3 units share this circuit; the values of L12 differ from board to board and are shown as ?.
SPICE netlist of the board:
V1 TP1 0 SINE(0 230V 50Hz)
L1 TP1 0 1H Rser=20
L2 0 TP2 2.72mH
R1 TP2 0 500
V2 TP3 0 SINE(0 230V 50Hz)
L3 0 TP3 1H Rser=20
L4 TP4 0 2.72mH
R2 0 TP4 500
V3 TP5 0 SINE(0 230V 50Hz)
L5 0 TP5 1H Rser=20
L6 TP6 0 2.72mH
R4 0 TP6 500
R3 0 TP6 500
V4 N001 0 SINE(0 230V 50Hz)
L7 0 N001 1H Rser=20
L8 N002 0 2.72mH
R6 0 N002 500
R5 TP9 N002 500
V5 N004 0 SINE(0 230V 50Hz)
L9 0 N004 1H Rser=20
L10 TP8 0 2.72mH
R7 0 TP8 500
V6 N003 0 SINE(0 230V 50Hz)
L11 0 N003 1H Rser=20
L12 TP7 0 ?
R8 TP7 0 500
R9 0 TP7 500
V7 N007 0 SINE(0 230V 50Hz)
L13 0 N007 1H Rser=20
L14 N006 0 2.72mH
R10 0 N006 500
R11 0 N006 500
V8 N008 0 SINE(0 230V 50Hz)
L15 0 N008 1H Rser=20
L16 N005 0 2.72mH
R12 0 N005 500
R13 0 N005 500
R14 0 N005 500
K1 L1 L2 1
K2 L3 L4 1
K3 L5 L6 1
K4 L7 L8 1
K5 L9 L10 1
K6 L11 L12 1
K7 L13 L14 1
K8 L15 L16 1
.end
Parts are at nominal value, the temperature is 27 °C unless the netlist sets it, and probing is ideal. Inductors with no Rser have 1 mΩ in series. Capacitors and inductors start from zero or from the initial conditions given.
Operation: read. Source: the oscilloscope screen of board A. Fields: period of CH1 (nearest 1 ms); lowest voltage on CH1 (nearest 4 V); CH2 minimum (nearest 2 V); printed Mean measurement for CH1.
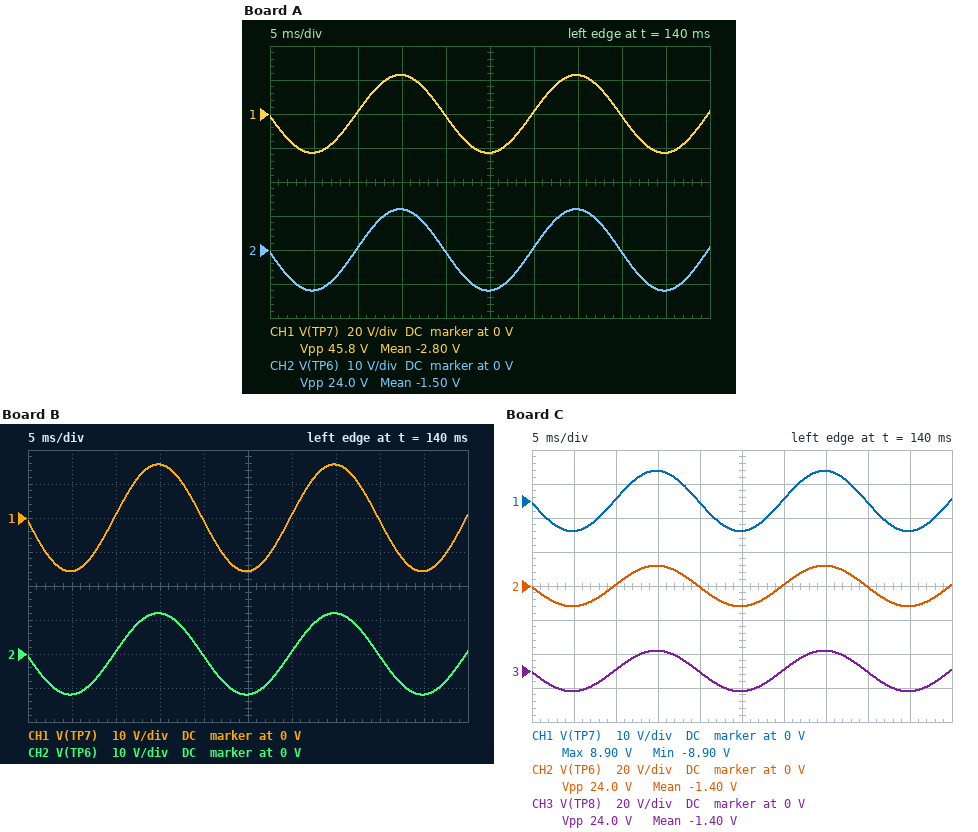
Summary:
20 ms
-24 V
-12 V
-2.80 V
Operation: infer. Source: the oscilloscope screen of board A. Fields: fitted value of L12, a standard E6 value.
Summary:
10 mH
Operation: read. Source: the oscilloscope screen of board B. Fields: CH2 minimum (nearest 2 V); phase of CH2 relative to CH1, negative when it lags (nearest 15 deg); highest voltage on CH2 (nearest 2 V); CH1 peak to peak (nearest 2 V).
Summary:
-12 V
0 deg
12 V
32 V
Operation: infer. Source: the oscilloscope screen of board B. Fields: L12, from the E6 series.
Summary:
4.7 mH
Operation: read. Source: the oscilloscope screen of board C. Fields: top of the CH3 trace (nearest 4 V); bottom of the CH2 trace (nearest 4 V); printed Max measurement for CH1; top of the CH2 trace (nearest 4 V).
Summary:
12 V
-12 V
8.90 V
12 V
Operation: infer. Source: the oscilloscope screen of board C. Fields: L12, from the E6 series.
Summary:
1.5 mH
